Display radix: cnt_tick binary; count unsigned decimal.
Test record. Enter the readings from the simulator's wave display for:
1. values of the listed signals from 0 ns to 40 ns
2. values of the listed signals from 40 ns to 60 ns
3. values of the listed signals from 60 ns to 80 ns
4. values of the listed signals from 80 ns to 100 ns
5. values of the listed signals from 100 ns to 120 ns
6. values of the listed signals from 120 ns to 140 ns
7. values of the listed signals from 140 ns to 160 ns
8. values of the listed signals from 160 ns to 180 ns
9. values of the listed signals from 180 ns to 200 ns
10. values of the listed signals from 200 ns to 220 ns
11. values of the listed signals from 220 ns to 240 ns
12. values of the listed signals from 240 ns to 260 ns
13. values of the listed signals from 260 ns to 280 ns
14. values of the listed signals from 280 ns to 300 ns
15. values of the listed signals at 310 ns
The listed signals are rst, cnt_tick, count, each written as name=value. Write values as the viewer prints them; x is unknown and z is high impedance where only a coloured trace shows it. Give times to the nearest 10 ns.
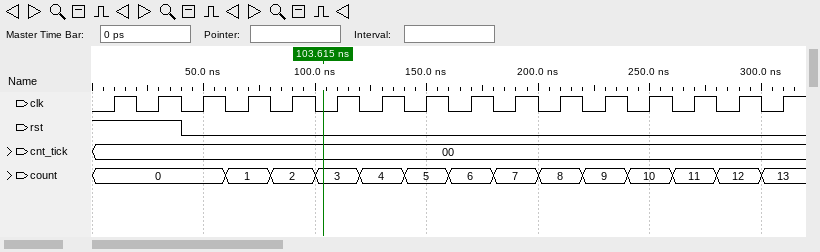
rst=1, cnt_tick=00, count=0
rst=0, cnt_tick=00, count=0
rst=0, cnt_tick=00, count=1
rst=0, cnt_tick=00, count=2
rst=0, cnt_tick=00, count=3
rst=0, cnt_tick=00, count=4
rst=0, cnt_tick=00, count=5
rst=0, cnt_tick=00, count=6
rst=0, cnt_tick=00, count=7
rst=0, cnt_tick=00, count=8
rst=0, cnt_tick=00, count=9
rst=0, cnt_tick=00, count=10
rst=0, cnt_tick=00, count=11
rst=0, cnt_tick=00, count=12
rst=0, cnt_tick=00, count=13
